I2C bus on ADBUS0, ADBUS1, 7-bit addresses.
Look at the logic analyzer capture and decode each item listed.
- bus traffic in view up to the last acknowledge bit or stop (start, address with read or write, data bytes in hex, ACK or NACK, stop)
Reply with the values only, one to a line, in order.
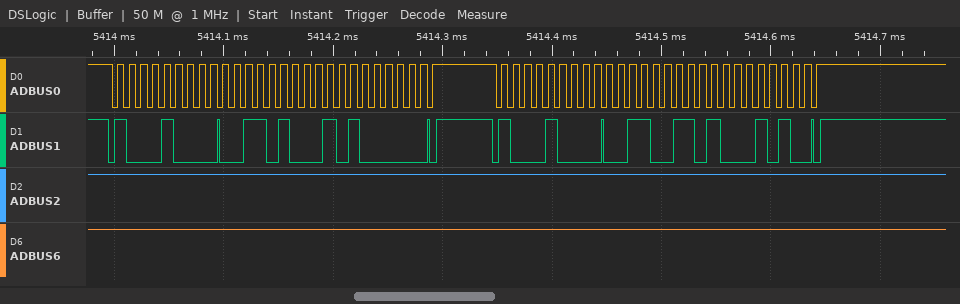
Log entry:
start, address 44 write ACK, 34 ACK, A0 ACK, stop, start, address 44 write ACK, 33 ACK, 8A ACK, stop
